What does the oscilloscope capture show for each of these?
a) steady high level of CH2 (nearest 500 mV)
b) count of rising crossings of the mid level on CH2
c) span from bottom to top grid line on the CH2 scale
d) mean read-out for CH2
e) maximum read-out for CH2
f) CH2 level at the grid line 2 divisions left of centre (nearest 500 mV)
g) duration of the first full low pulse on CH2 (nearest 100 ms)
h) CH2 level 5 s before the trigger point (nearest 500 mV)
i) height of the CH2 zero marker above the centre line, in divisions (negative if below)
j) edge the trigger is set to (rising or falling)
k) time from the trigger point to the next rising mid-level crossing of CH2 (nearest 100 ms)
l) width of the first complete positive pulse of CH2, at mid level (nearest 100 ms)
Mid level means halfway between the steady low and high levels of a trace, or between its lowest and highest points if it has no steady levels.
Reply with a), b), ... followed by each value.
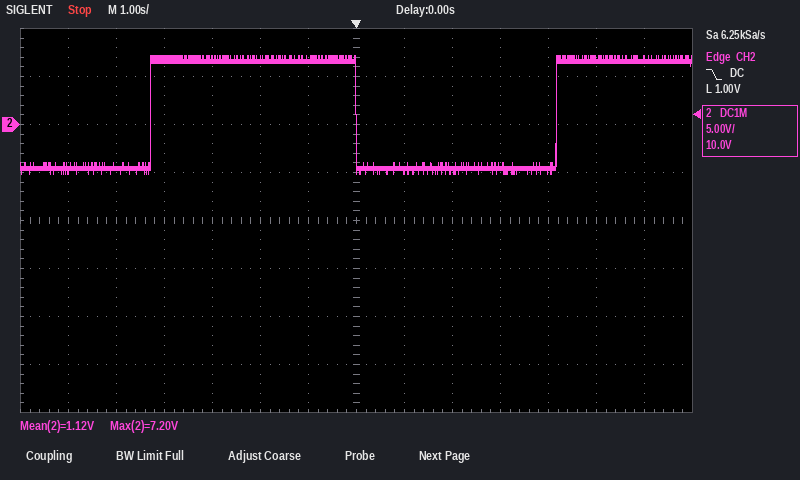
a) 7.0 V
b) 2
c) 40 V
d) 1.12 V
e) 7.20 V
f) 7.0 V
g) 4.2 s
h) -4.5 V
i) +2.0 div
j) falling
k) 4.2 s
l) 4.3 s
